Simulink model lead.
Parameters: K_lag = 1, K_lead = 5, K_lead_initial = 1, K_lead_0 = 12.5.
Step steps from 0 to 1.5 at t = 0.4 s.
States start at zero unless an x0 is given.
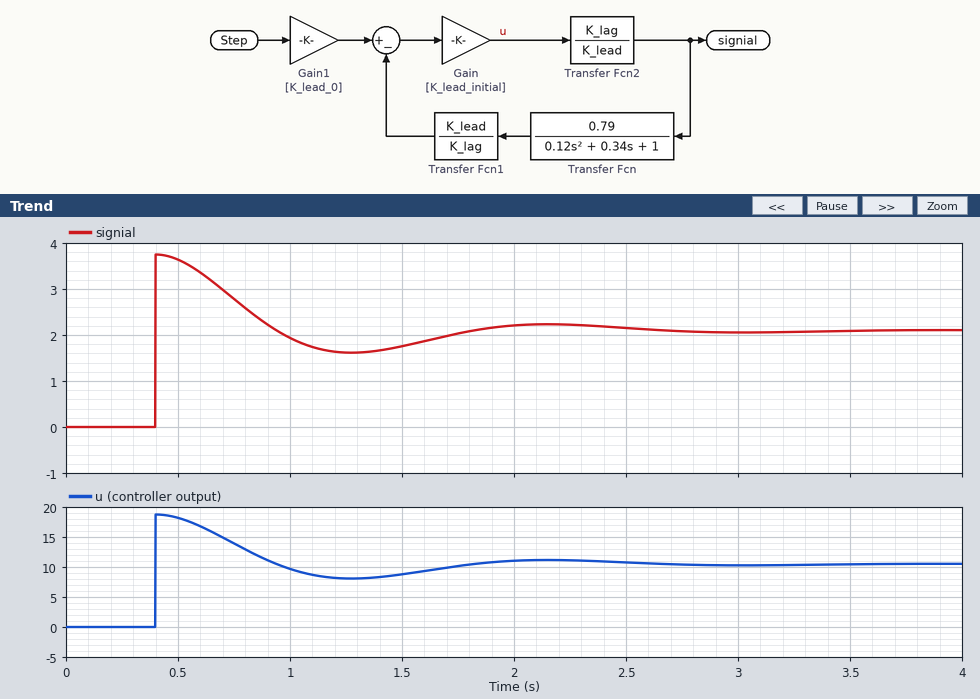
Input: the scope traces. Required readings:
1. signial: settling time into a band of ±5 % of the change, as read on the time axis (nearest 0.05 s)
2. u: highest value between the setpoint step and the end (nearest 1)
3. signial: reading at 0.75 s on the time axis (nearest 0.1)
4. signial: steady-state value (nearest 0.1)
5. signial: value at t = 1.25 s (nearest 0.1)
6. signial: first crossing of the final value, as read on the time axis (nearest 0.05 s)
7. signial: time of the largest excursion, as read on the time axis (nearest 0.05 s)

2.35 s
19
2.8
2.1
1.6
0.40 s
0.40 s
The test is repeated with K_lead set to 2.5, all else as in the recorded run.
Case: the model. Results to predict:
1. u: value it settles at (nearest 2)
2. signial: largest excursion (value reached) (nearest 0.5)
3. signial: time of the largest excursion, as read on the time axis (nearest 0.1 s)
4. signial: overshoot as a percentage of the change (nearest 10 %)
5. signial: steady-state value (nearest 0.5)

10
7.5
0.4 s
80 %
4.0
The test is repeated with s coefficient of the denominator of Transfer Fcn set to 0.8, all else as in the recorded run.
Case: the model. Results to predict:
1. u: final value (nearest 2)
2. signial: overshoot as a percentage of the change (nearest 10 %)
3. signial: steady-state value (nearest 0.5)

10
80 %
2.0
